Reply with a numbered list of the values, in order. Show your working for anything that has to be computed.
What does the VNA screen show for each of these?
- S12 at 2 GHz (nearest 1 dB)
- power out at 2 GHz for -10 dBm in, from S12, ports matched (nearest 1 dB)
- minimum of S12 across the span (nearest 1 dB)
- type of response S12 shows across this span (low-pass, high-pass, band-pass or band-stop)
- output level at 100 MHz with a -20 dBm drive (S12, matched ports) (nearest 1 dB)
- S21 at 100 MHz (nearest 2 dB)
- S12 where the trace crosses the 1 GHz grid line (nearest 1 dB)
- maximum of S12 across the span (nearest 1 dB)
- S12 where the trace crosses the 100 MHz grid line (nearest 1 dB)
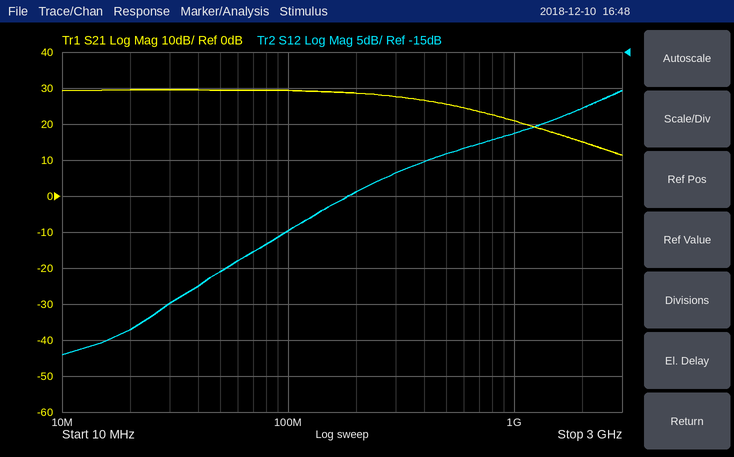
1. -23 dB
2. -10 dBm + (-23 dB) = -33 dBm
3. -57 dB
4. high-pass
5. -20 dBm + (-40 dB) = -60 dBm
6. 30 dB
7. -26 dB
8. -20 dB
9. -40 dB
